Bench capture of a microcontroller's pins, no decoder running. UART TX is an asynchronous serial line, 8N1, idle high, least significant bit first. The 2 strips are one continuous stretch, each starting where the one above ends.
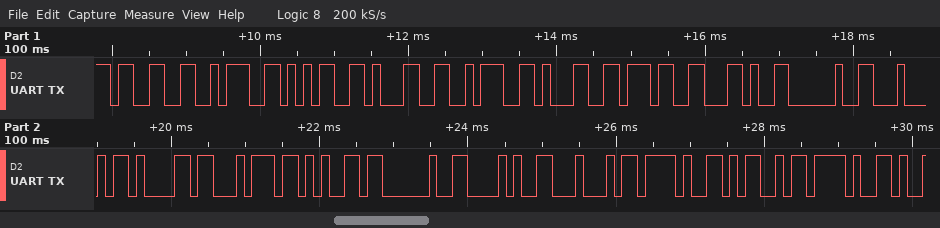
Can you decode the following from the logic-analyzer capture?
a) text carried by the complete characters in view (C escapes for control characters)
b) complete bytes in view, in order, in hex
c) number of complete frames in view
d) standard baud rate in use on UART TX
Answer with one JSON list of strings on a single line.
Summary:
["\"3:51:17, Date (D/M/\"", "33 3A 35 31 3A 31 37 2C 20 44 61 74 65 20 28 44 2F 4D 2F", "19", "9600 baud"]
